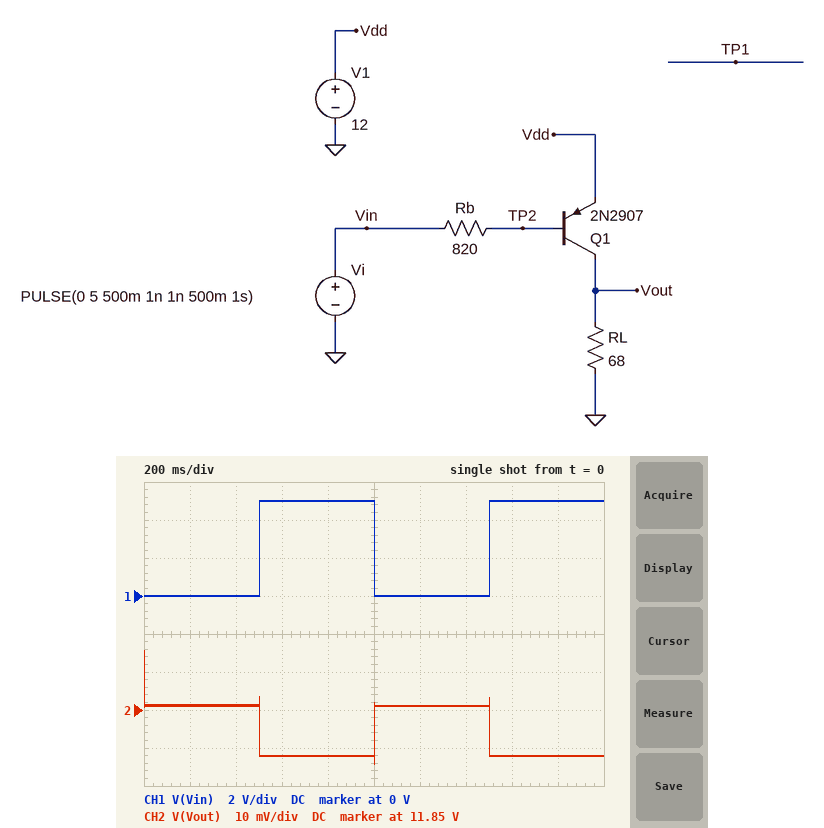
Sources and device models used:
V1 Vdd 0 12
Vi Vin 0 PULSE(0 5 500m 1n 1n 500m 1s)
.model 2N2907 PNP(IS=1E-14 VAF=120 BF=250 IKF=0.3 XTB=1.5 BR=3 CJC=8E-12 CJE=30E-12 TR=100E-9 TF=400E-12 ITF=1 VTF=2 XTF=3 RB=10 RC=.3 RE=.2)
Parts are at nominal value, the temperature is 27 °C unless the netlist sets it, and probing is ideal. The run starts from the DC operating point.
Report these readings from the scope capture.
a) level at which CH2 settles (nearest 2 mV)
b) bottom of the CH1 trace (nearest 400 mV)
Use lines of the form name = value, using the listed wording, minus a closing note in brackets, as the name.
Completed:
level at which CH2 settles = 11.838 V
bottom of the CH1 trace = 0 V
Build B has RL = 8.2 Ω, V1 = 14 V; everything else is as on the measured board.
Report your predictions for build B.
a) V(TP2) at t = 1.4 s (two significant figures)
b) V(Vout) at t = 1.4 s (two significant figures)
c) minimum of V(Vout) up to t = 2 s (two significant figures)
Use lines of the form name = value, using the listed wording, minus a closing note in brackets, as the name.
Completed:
V(TP2) at t = 1.4 s = 13 V
V(Vout) at t = 1.4 s = 8.0 V
minimum of V(Vout) up to t = 2 s = 6.2 V
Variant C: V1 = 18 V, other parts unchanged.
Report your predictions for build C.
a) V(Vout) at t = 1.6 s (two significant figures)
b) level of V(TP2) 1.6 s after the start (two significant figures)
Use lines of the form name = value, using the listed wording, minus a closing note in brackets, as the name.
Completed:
V(Vout) at t = 1.6 s = 18 V
level of V(TP2) 1.6 s after the start = 17 V
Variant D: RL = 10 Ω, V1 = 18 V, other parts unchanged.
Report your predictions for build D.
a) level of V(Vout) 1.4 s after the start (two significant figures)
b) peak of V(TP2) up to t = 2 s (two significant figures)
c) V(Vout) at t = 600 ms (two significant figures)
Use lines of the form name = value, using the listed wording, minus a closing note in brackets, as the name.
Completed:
level of V(Vout) 1.4 s after the start = 11 V
peak of V(TP2) up to t = 2 s = 17 V
V(Vout) at t = 600 ms = 9.5 V
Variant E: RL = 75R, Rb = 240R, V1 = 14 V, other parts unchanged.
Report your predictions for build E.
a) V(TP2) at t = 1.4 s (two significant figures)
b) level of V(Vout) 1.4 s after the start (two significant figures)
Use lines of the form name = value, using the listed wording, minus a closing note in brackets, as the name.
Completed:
V(TP2) at t = 1.4 s = 13 V
level of V(Vout) 1.4 s after the start = 14 V
